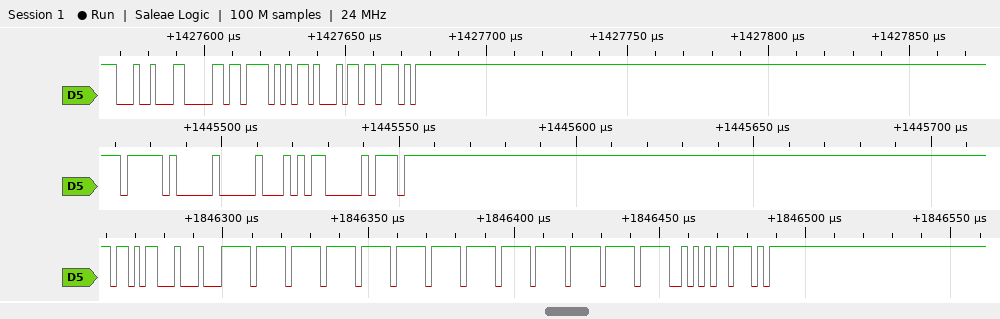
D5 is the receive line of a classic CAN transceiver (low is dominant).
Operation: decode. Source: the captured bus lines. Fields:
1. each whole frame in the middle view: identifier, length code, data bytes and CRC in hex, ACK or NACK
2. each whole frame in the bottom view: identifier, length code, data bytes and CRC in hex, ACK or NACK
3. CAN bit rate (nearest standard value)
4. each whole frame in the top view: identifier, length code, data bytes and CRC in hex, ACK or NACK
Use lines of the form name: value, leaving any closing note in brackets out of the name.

each whole frame in the middle view: identifier, length code, data bytes and CRC in hex, ACK or NACK: ID 7E0, DLC 0, CRC 2B03, ACK
each whole frame in the bottom view: identifier, length code, data bytes and CRC in hex, ACK or NACK: ID 6B1, DLC 8, data FF FF FF FF FF FF FF FF, CRC 556E, ACK
CAN bit rate: 500 kbit/s
each whole frame in the top view: identifier, length code, data bytes and CRC in hex, ACK or NACK: ID 123, DLC 2, data DE AD, CRC 0B6E, ACK
